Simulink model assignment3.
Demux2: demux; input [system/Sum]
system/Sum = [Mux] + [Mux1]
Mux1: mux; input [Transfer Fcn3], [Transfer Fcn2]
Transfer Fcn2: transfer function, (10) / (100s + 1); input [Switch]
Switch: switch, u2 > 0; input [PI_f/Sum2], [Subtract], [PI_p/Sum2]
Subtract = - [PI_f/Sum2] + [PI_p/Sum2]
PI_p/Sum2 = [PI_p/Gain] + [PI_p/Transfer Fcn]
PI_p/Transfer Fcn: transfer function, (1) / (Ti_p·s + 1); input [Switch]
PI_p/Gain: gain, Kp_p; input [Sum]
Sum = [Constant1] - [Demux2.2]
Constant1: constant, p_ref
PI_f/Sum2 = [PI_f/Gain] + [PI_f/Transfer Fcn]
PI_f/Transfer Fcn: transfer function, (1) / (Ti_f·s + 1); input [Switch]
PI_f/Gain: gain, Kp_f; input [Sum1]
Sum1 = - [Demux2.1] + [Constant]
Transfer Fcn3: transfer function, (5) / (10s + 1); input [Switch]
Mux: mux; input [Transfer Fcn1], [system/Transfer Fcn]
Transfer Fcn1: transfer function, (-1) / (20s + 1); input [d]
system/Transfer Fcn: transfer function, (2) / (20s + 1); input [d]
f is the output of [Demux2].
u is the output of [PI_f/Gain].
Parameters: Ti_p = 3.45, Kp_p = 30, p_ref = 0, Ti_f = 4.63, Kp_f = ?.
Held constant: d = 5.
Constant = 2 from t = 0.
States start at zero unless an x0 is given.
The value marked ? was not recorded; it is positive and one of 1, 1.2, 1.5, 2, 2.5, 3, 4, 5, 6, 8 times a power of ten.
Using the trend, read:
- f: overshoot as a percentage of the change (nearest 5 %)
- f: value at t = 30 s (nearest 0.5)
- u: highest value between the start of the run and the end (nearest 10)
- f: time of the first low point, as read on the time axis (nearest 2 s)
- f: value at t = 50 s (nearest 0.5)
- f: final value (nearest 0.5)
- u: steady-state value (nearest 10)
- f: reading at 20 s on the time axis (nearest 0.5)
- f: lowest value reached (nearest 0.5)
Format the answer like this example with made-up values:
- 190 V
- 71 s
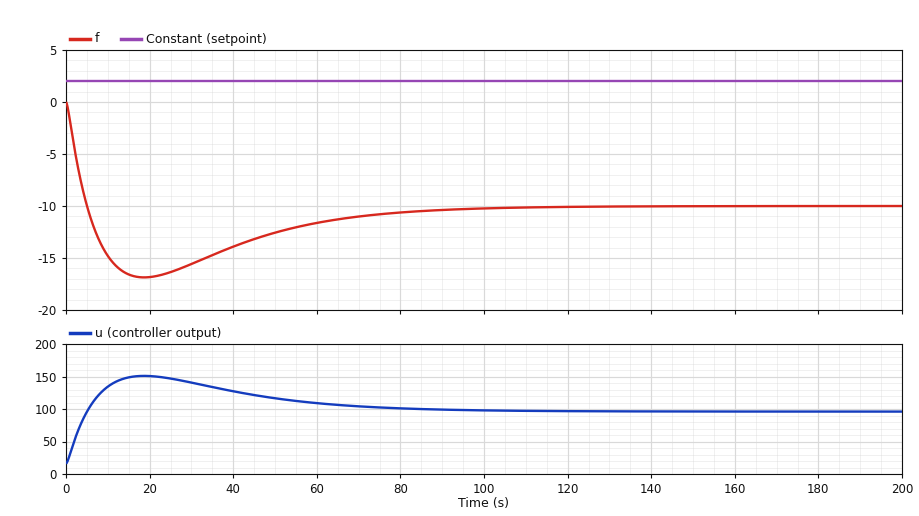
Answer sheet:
- 70 %
- -15.5
- 150
- 18 s
- -12.5
- -10.0
- 100
- -17.0
- -17.0
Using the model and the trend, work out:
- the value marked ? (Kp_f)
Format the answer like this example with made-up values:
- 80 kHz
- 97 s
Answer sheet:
- 8
